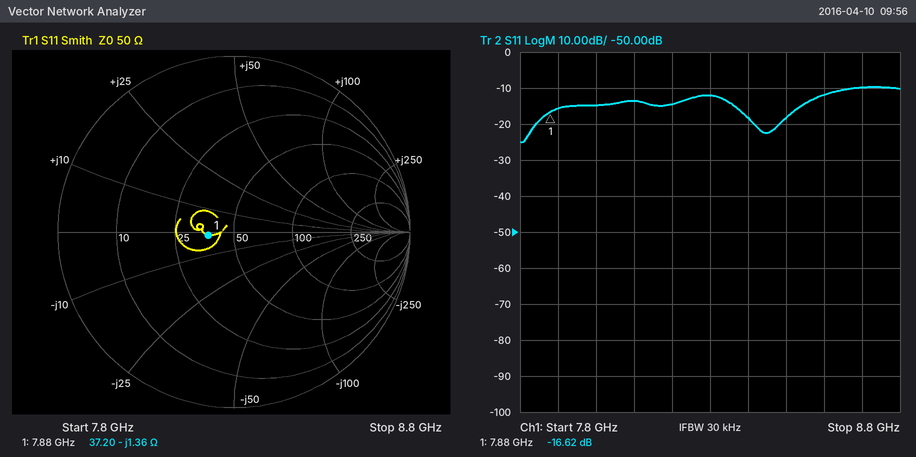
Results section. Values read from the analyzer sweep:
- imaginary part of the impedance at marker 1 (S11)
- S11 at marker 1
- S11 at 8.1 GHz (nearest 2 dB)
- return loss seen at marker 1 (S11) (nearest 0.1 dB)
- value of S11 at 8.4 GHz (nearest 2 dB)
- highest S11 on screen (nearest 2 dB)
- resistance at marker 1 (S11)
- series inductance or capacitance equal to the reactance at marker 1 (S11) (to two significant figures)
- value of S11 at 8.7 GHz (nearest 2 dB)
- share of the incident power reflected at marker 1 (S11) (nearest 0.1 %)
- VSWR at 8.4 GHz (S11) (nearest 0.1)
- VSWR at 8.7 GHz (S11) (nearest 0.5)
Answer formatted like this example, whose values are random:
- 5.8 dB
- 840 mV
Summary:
- -1.36 Ω
- -16.62 dB
- -14 dB
- 16.6 dB
- -18 dB
- -10 dB
- 37.20 Ω
- 15 pF
- -10 dB
- 2.2 %
- 1.3
- 2.0
